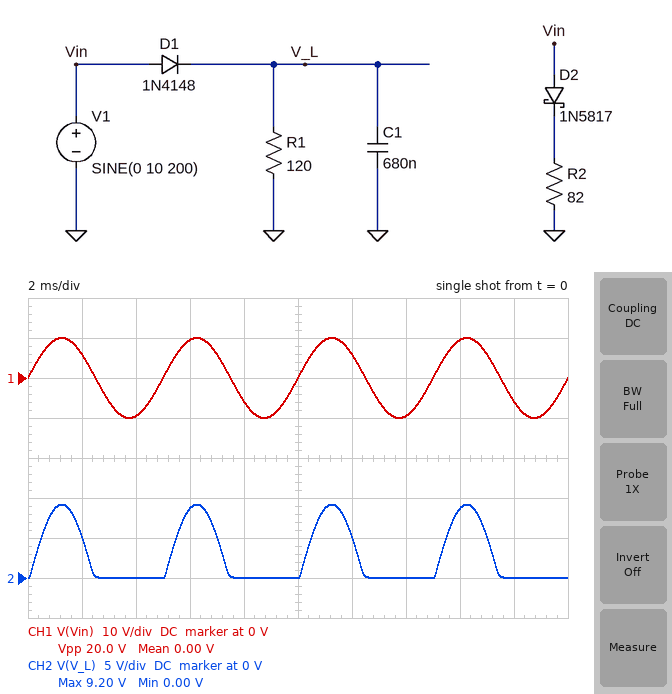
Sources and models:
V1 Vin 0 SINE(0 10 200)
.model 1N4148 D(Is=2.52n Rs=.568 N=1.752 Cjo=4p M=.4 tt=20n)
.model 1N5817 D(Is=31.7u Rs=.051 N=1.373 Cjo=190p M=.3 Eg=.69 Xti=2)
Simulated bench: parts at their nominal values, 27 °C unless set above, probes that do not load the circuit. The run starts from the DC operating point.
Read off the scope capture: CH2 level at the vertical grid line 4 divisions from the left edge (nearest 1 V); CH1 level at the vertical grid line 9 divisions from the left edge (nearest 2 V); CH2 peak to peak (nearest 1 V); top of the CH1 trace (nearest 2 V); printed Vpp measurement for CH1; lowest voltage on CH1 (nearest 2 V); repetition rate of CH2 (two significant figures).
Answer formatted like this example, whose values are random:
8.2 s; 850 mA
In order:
0 V; -6 V; 9 V; 10 V; 20.0 V; -10 V; 200 Hz
